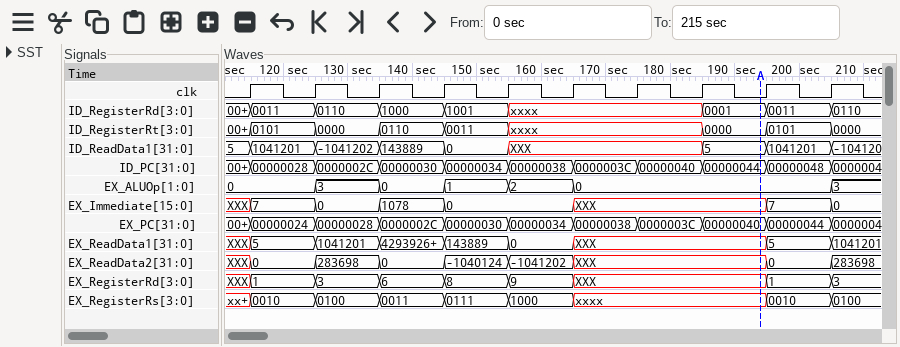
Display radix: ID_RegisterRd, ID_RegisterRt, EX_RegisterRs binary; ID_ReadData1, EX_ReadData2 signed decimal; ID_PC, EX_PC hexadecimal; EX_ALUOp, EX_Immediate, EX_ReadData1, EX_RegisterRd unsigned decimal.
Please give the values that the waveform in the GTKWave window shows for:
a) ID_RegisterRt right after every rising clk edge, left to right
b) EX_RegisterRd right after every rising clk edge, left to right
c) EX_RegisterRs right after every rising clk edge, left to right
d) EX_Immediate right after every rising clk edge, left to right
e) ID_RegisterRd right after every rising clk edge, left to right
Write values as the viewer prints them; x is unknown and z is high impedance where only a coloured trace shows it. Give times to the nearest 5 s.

0101, 0000, 0110, 0011, xxxx, xxxx, xxxx, 0000, 0101, 0000
1, 3, 6, 8, 9, XXX, XXX, XXX, 1, 3
0010, 0100, 0011, 0111, 1000, xxxx, xxxx, xxxx, 0010, 0100
7, 0, 1078, 0, 0, XXX, XXX, XXX, 7, 0
0011, 0110, 1000, 1001, xxxx, xxxx, xxxx, 0001, 0011, 0110
